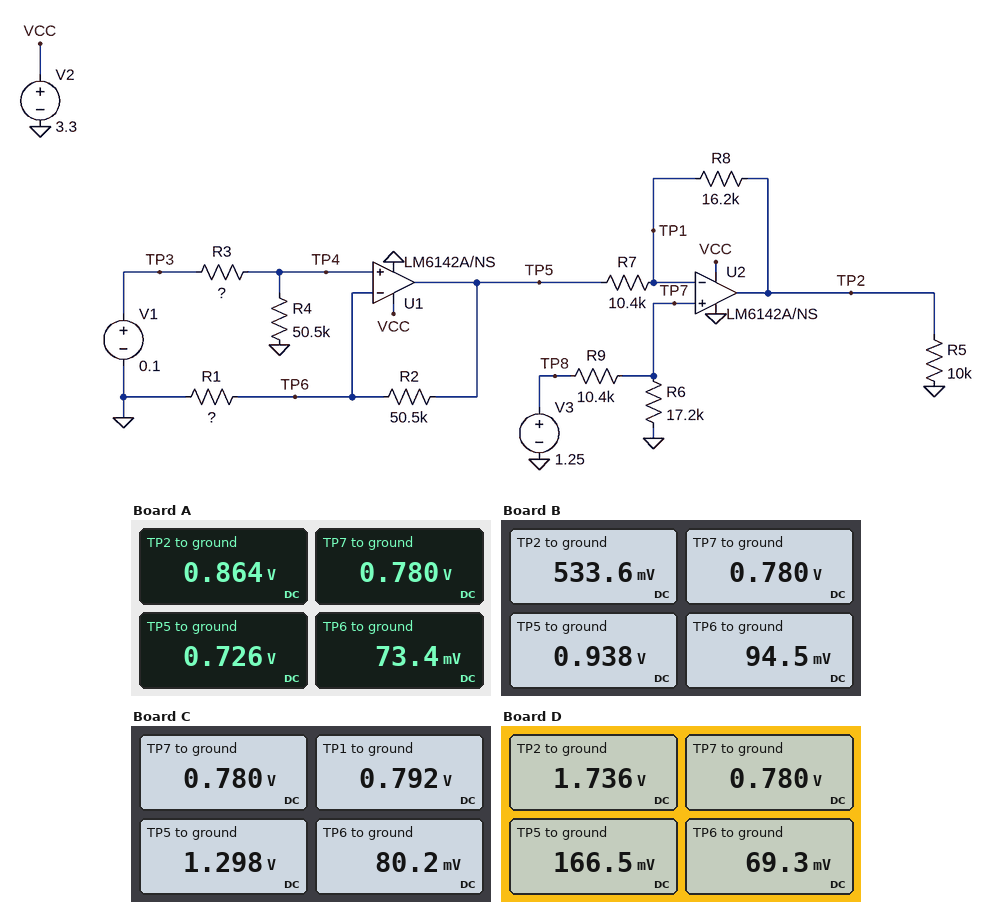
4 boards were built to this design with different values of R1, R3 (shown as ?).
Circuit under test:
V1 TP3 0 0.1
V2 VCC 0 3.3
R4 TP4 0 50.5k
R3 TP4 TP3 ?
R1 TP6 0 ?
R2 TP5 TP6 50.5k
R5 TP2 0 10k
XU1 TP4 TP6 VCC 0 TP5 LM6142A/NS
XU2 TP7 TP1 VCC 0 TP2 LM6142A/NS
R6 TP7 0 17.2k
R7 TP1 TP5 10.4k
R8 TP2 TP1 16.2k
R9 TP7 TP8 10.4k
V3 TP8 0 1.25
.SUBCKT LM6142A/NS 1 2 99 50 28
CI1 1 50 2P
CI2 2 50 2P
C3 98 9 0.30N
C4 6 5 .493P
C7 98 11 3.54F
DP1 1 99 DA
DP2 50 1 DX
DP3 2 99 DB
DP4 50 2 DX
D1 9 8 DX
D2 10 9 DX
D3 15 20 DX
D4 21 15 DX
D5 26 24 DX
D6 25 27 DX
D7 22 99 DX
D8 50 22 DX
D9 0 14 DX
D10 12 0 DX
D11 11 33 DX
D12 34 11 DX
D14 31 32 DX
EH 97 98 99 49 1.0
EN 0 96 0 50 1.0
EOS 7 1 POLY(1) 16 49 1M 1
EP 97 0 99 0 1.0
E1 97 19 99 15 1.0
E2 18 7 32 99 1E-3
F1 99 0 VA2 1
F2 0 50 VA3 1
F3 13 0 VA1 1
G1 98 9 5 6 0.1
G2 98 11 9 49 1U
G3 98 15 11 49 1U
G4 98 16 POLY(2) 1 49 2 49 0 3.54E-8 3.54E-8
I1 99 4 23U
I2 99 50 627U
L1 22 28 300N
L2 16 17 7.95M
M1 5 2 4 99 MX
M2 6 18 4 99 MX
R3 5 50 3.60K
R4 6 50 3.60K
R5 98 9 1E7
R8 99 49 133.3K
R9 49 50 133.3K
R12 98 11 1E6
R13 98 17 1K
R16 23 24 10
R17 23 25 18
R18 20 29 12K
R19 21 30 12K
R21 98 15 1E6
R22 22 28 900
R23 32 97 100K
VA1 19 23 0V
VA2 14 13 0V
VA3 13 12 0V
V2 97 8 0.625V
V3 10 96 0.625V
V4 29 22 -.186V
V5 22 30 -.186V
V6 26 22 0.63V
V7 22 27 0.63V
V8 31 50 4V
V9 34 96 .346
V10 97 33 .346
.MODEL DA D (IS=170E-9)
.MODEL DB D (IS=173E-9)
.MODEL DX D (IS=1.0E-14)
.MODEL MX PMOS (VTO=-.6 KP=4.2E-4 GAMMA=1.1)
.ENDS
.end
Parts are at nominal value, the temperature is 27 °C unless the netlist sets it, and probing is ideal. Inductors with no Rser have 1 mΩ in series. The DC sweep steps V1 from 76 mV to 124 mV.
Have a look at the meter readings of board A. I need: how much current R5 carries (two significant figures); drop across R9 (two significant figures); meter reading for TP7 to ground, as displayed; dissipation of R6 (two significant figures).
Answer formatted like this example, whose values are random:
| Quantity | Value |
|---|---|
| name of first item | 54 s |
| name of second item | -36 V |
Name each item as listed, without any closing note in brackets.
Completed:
| Quantity | Value |
|---|---|
| how much current R5 carries | 86 µA |
| drop across R9 | 470 mV |
| meter reading for TP7 to ground, as displayed | 0.780 V |
| dissipation of R6 | 35 µW |
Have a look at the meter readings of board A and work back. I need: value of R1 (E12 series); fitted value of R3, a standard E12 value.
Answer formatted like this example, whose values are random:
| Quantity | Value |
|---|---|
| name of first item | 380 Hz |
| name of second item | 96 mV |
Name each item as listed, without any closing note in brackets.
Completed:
| Quantity | Value |
|---|---|
| value of R1 | 5.6 kΩ |
| fitted value of R3, a standard E12 value | 22 kΩ |
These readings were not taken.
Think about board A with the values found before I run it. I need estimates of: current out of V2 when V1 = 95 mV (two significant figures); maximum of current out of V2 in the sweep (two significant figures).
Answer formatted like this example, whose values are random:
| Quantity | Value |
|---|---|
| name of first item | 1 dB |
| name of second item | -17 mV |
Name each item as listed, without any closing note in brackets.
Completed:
| Quantity | Value |
|---|---|
| current out of V2 when V1 = 95 mV | 1.4 mA |
| maximum of current out of V2 in the sweep | 1.5 mA |
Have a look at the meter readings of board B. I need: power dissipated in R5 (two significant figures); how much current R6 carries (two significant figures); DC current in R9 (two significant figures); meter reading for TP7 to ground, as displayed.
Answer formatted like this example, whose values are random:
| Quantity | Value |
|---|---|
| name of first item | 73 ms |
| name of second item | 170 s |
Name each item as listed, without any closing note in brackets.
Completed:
| Quantity | Value |
|---|---|
| power dissipated in R5 | 28 µW |
| how much current R6 carries | 45 µA |
| DC current in R9 | 45 µA |
| meter reading for TP7 to ground, as displayed | 0.780 V |
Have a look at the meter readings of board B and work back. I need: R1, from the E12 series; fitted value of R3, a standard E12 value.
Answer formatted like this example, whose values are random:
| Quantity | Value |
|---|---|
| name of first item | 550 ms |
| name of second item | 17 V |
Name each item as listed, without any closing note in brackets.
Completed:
| Quantity | Value |
|---|---|
| R1, from the E12 series | 5.6 kΩ |
| fitted value of R3, a standard E12 value | 3.9 kΩ |
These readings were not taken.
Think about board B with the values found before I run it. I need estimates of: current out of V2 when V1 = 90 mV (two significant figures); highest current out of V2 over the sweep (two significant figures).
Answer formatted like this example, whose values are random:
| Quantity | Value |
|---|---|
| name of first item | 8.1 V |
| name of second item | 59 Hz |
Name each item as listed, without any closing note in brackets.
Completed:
| Quantity | Value |
|---|---|
| current out of V2 when V1 = 90 mV | 1.4 mA |
| highest current out of V2 over the sweep | 1.4 mA |
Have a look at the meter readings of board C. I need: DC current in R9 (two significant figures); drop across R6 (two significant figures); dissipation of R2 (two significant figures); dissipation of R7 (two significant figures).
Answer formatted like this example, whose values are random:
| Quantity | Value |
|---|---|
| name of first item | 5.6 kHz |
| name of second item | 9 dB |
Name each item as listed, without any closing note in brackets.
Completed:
| Quantity | Value |
|---|---|
| DC current in R9 | 45 µA |
| drop across R6 | 780 mV |
| dissipation of R2 | 29 µW |
| dissipation of R7 | 25 µW |
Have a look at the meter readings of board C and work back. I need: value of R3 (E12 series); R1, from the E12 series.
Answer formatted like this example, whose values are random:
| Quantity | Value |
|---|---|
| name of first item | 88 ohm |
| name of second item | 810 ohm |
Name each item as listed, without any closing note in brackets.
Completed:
| Quantity | Value |
|---|---|
| value of R3 | 15 kΩ |
| R1, from the E12 series | 3.3 kΩ |
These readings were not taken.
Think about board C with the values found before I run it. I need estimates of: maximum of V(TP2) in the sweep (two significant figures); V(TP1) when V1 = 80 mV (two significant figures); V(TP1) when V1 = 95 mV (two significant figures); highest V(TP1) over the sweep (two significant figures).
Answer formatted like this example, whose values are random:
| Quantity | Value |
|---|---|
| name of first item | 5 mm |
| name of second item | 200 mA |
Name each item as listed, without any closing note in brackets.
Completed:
| Quantity | Value |
|---|---|
| maximum of V(TP2) in the sweep | 440 mV |
| V(TP1) when V1 = 80 mV | 780 mV |
| V(TP1) when V1 = 95 mV | 780 mV |
| highest V(TP1) over the sweep | 960 mV |
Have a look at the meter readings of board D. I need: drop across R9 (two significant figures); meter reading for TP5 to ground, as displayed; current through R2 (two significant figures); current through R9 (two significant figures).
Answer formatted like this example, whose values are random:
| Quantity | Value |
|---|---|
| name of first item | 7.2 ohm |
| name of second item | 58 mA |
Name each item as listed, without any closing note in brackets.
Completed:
| Quantity | Value |
|---|---|
| drop across R9 | 470 mV |
| meter reading for TP5 to ground, as displayed | 166.5 mV |
| current through R2 | 1.9 µA |
| current through R9 | 45 µA |
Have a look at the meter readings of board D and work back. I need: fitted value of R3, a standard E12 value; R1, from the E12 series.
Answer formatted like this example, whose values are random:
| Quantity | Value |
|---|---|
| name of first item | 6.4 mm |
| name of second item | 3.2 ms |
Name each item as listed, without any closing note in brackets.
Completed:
| Quantity | Value |
|---|---|
| fitted value of R3, a standard E12 value | 27 kΩ |
| R1, from the E12 series | 33 kΩ |
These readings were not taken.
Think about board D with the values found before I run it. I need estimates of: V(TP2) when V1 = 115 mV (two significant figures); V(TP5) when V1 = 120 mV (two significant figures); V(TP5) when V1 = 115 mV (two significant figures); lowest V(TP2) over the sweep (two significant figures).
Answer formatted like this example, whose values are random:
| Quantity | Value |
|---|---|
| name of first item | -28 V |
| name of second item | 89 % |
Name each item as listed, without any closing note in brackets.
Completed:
| Quantity | Value |
|---|---|
| V(TP2) when V1 = 115 mV | 1.7 V |
| V(TP5) when V1 = 120 mV | 200 mV |
| V(TP5) when V1 = 115 mV | 190 mV |
| lowest V(TP2) over the sweep | 1.7 V |
